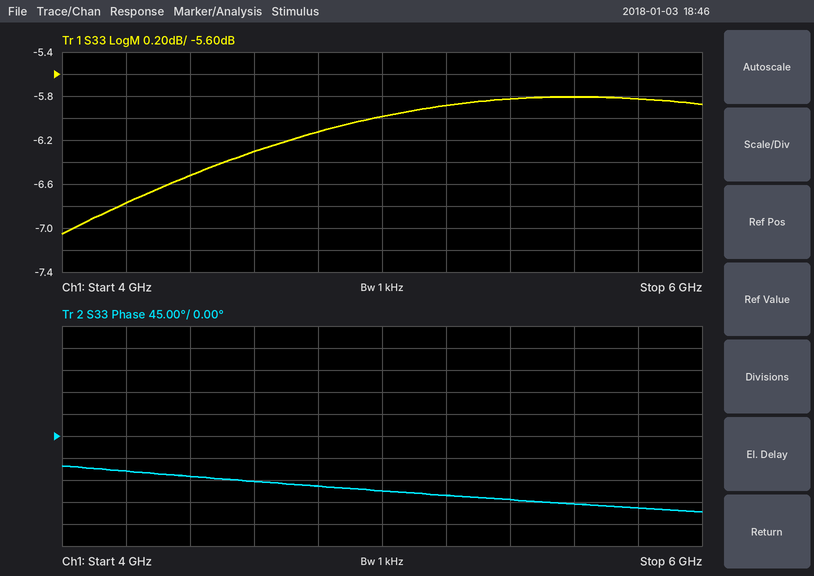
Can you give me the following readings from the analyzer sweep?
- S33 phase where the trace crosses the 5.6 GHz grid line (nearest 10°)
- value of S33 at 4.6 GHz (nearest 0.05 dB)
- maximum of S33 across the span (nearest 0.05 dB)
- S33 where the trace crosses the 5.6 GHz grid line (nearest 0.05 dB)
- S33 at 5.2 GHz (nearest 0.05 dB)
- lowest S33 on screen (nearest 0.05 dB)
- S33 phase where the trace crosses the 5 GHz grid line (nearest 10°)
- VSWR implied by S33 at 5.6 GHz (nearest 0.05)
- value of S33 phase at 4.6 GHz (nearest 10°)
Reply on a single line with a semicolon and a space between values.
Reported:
-140°; -6.30 dB; -5.80 dB; -5.80 dB; -5.90 dB; -7.05 dB; -110°; 3.10; -90°
